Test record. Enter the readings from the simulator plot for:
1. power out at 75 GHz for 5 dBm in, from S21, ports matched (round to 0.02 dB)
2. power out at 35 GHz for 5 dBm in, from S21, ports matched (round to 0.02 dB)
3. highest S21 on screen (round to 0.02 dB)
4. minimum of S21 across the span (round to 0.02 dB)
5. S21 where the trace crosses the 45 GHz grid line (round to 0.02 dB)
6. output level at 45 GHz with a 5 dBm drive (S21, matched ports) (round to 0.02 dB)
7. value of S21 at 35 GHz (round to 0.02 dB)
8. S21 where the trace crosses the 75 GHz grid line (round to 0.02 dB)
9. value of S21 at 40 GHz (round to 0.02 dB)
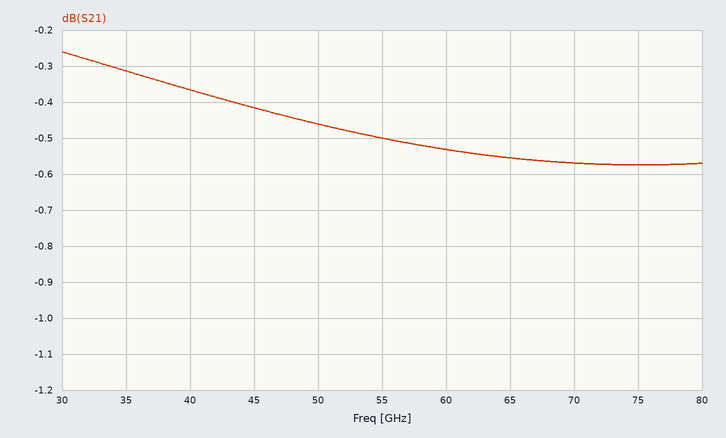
4.42 dBm
4.68 dBm
-0.26 dB
-0.58 dB
-0.42 dB
4.58 dBm
-0.32 dB
-0.58 dB
-0.36 dB
